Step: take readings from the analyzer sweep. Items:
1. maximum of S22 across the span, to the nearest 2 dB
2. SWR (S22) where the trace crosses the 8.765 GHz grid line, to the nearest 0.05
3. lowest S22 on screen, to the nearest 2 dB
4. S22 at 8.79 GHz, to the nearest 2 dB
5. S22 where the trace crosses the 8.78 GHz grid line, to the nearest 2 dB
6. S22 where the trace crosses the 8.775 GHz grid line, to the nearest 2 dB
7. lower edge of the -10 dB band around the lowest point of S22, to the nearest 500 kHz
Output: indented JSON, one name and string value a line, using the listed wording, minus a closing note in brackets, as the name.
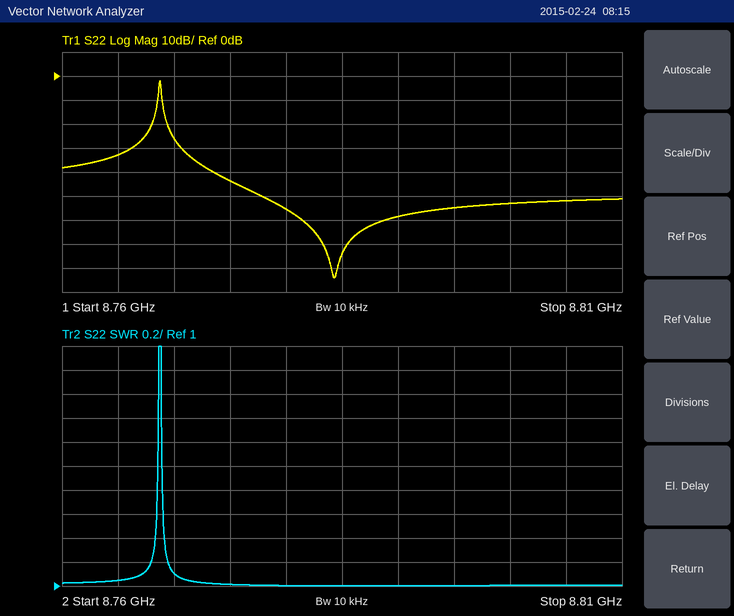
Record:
{
  "maximum of S22 across the span, to the nearest 2 dB": "-2 dB",
  "SWR (S22) where the trace crosses the 8.765 GHz grid line, to the nearest 0.05": "1.05",
  "lowest S22 on screen, to the nearest 2 dB": "-84 dB",
  "S22 at 8.79 GHz, to the nearest 2 dB": "-58 dB",
  "S22 where the trace crosses the 8.78 GHz grid line, to the nearest 2 dB": "-56 dB",
  "S22 where the trace crosses the 8.775 GHz grid line, to the nearest 2 dB": "-44 dB",
  "lower edge of the -10 dB band around the lowest point of S22, to the nearest 500 kHz": "8.7690 GHz"
}
